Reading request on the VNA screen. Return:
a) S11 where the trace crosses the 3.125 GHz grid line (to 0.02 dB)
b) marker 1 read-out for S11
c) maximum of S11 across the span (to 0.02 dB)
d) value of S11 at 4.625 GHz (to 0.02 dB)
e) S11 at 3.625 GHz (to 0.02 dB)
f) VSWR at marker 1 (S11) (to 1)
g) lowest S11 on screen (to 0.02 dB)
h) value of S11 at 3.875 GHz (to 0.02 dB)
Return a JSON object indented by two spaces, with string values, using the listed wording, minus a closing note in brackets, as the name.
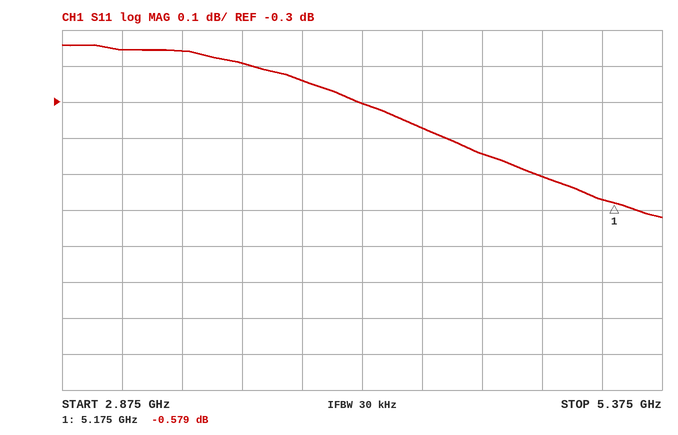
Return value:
{
  "S11 where the trace crosses the 3.125 GHz grid line": "-0.16 dB",
  "marker 1 read-out for S11": "-0.579 dB",
  "maximum of S11 across the span": "-0.14 dB",
  "value of S11 at 4.625 GHz": "-0.44 dB",
  "S11 at 3.625 GHz": "-0.20 dB",
  "VSWR at marker 1 (S11)": "30",
  "lowest S11 on screen": "-0.62 dB",
  "value of S11 at 3.875 GHz": "-0.24 dB"
}
